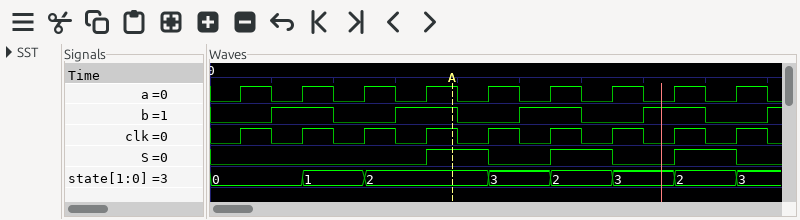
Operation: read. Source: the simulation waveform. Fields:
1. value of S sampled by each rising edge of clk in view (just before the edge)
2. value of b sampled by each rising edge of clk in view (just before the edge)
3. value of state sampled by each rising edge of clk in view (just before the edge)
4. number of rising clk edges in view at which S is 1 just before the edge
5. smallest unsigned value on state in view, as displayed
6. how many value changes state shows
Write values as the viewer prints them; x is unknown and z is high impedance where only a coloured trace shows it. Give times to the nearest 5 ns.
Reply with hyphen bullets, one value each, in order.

- 0 0 0 0 1 0 1 0 1
- 0 1 0 1 0 1 0 1 0
- 0, 0, 1, 2, 2, 3, 2, 3, 2
- 3
- 0
- 7
